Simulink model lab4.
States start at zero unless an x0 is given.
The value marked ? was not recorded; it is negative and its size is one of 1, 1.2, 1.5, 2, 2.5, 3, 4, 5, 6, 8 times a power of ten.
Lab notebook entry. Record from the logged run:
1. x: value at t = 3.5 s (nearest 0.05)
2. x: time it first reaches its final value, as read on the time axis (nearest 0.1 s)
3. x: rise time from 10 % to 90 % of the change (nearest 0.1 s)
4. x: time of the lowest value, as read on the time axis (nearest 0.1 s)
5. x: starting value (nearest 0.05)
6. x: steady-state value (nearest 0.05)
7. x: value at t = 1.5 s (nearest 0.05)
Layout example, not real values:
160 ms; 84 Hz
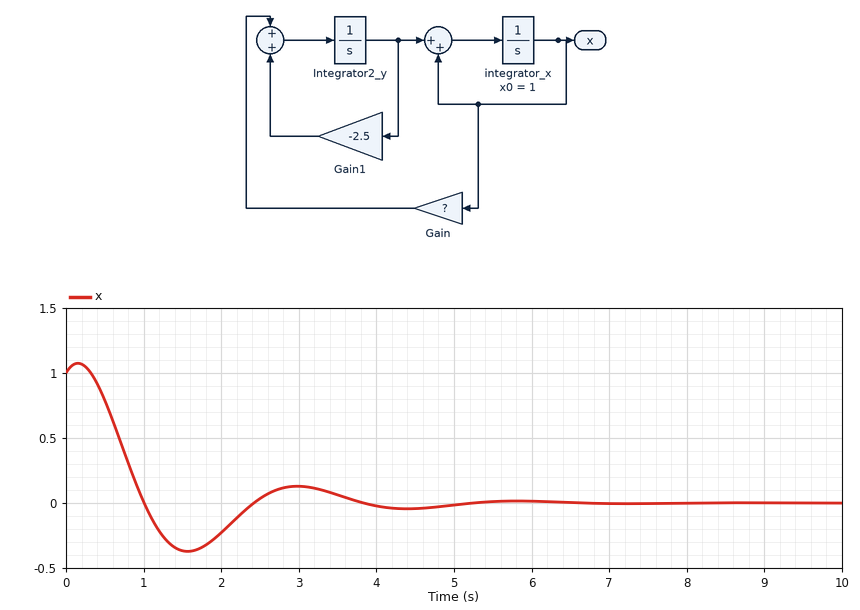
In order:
0.05; 1.0 s; 0.5 s; 1.6 s; 1.00; 0.00; -0.35
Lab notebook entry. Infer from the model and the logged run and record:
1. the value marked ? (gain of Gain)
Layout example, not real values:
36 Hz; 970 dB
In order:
-8
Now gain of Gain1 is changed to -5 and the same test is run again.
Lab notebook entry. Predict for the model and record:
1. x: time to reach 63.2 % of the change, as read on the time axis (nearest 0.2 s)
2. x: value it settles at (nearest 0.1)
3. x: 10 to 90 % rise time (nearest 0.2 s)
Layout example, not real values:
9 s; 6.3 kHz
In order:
1.6 s; 0.0; 2.4 s
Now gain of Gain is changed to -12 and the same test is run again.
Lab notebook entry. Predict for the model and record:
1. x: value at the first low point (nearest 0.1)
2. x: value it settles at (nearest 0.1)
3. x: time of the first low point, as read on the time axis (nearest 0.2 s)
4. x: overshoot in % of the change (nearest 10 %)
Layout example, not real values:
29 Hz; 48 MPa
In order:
-0.5; 0.0; 1.2 s; 50 %
